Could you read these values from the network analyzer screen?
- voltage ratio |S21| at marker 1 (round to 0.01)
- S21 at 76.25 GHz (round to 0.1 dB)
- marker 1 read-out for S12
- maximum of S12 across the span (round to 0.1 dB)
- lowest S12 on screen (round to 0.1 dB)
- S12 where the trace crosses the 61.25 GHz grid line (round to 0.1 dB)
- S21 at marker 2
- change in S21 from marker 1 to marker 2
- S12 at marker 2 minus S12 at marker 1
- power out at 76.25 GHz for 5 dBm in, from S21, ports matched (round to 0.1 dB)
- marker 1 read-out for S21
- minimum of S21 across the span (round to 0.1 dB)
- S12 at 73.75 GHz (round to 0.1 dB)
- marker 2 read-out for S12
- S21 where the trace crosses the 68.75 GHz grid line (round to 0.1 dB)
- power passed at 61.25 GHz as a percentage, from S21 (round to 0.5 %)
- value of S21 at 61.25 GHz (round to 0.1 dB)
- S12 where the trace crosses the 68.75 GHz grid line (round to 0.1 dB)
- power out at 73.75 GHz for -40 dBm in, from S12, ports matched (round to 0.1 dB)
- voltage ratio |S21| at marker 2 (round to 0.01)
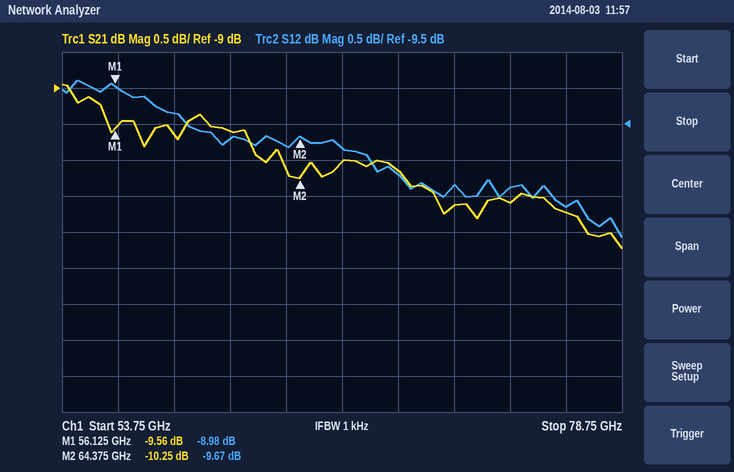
0.33
-10.7 dB
-8.98 dB
-8.9 dB
-11.1 dB
-9.7 dB
-10.25 dB
-0.69 dB
-0.69 dB
-5.7 dBm
-9.56 dB
-11.2 dB
-10.4 dB
-9.67 dB
-10.1 dB
11.0 %
-9.6 dB
-10.2 dB
-50.4 dBm
0.31
